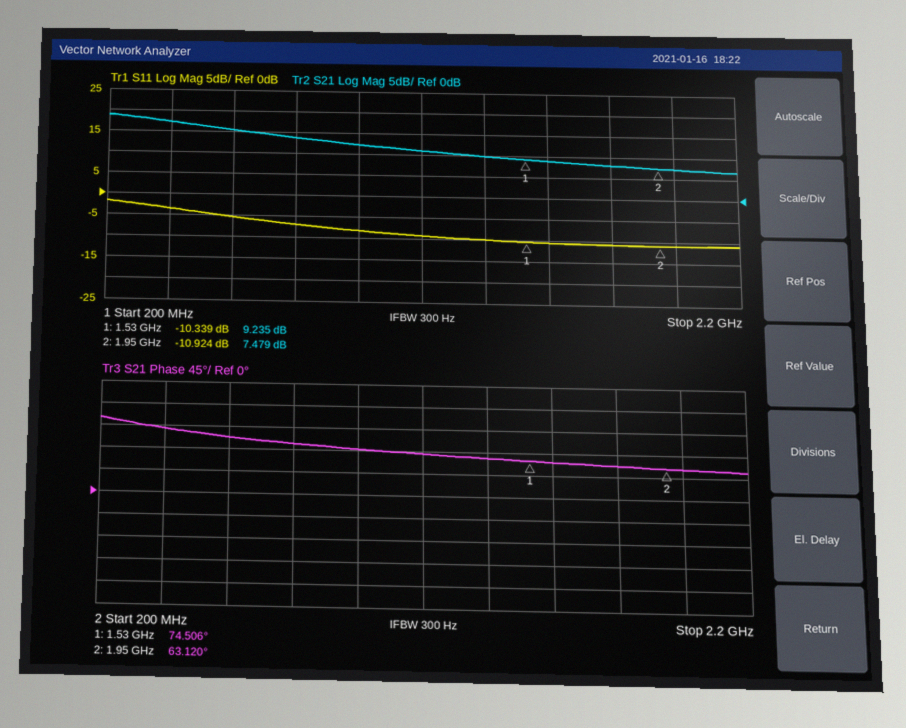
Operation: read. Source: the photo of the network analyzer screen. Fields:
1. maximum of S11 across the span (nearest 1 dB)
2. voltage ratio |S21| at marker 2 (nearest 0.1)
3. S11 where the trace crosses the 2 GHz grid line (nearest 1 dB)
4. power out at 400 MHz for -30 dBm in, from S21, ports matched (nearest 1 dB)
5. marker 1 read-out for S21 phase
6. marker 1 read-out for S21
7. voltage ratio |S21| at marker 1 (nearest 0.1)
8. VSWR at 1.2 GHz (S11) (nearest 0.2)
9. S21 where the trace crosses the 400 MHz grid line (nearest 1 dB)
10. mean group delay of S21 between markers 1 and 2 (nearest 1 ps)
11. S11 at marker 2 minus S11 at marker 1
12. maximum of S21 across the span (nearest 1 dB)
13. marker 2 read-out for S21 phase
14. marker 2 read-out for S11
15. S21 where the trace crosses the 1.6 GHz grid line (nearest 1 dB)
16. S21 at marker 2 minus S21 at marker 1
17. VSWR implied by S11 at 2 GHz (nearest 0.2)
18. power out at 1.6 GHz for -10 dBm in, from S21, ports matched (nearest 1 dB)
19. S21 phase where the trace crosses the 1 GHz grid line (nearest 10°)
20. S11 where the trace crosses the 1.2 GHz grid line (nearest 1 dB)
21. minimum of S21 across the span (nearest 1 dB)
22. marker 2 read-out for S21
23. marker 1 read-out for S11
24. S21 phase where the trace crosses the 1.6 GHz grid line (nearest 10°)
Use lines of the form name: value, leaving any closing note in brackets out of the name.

maximum of S11 across the span: -2 dB
voltage ratio |S21| at marker 2: 2.4
S11 where the trace crosses the 2 GHz grid line: -11 dB
power out at 400 MHz for -30 dBm in, from S21, ports matched: -13 dBm
marker 1 read-out for S21 phase: 74.506°
marker 1 read-out for S21: 9.235 dB
voltage ratio |S21| at marker 1: 2.9
VSWR at 1.2 GHz (S11): 2.0
S21 where the trace crosses the 400 MHz grid line: 17 dB
mean group delay of S21 between markers 1 and 2: 75 ps
S11 at marker 2 minus S11 at marker 1: -0.585 dB
maximum of S21 across the span: 19 dB
marker 2 read-out for S21 phase: 63.120°
marker 2 read-out for S11: -10.924 dB
S21 where the trace crosses the 1.6 GHz grid line: 9 dB
S21 at marker 2 minus S21 at marker 1: -1.756 dB
VSWR implied by S11 at 2 GHz: 1.8
power out at 1.6 GHz for -10 dBm in, from S21, ports matched: -1 dBm
S21 phase where the trace crosses the 1 GHz grid line: 90°
S11 where the trace crosses the 1.2 GHz grid line: -9 dB
minimum of S21 across the span: 7 dB
marker 2 read-out for S21: 7.479 dB
marker 1 read-out for S11: -10.339 dB
S21 phase where the trace crosses the 1.6 GHz grid line: 70°
